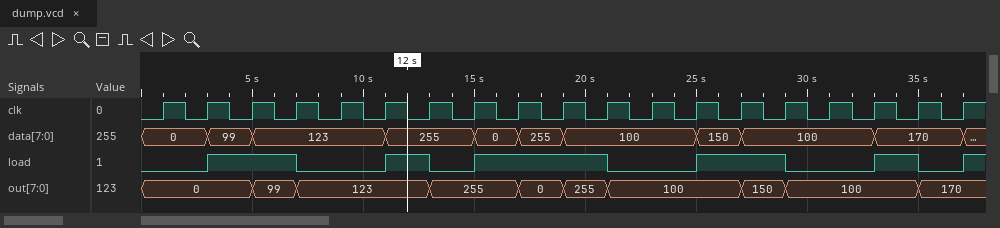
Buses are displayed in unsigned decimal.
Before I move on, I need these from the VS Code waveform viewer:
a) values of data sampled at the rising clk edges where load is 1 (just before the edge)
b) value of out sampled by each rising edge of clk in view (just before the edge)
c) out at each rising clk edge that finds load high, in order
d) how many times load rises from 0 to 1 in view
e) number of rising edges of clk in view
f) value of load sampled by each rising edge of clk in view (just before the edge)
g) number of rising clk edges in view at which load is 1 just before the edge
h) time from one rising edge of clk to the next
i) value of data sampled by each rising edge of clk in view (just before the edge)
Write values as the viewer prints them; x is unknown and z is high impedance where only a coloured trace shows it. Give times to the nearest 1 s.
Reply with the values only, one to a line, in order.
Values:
99, 123, 255, 0, 255, 100, 150, 100, 170
0, 0, 0, 99, 123, 123, 123, 255, 255, 0, 255, 100, 100, 100, 150, 100, 100, 100, 170
0, 99, 123, 255, 0, 255, 100, 150, 100
6
19
0 0 1 1 0 0 1 0 1 1 1 0 0 1 1 0 0 1 0
9
2 s
0, 0, 99, 123, 123, 123, 255, 255, 0, 255, 100, 100, 100, 150, 100, 100, 100, 170, 170
